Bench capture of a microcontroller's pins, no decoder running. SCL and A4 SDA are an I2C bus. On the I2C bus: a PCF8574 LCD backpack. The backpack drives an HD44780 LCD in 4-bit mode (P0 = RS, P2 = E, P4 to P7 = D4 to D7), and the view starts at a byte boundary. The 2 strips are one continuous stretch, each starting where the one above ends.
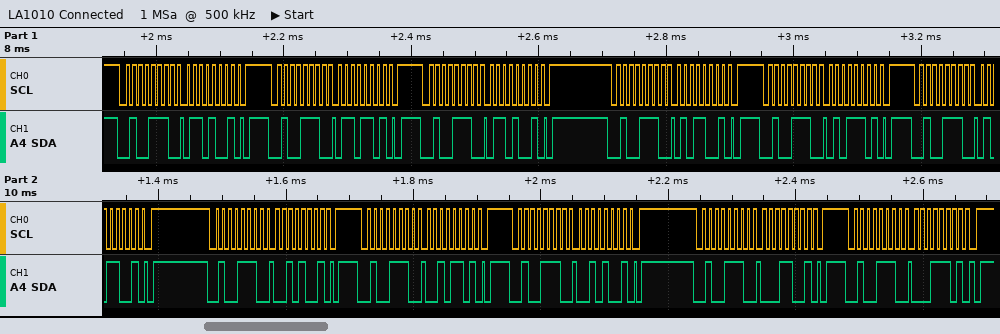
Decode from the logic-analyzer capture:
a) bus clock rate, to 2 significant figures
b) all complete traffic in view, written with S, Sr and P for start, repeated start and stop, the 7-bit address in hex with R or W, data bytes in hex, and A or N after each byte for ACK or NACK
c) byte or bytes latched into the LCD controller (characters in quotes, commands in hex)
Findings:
100 kHz
S 27W A 69 A P S 27W A 6D A P S 27W A 69 A P S 27W A 59 A P S 27W A 5D A P S 27W A 59 A P S 27W A 29 A P S 27W A 2D A P S 27W A 29 A P S 27W A 19 A P S 27W A 1D A P
'e'
